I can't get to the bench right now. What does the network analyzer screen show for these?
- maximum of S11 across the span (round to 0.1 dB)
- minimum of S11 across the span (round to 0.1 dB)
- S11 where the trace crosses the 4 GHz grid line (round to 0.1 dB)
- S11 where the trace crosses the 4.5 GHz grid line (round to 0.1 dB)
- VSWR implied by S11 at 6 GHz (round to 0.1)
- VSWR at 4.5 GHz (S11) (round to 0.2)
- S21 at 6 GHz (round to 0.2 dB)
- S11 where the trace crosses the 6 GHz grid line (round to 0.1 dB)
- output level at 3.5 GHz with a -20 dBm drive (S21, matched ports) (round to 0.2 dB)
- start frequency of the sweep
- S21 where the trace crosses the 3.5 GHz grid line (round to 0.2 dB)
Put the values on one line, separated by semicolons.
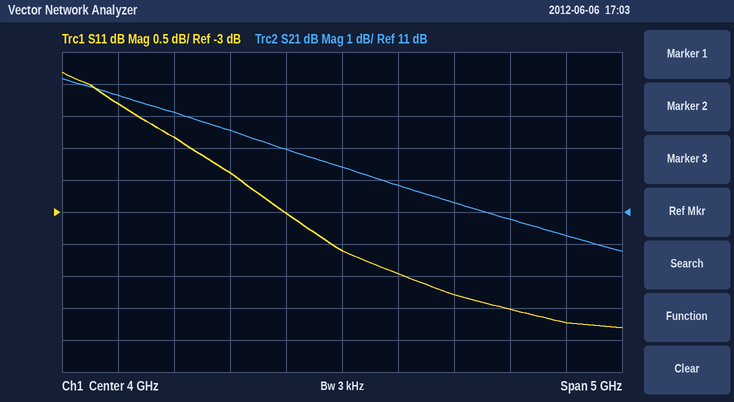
-0.8 dB; -4.8 dB; -3.6 dB; -4.0 dB; 3.8; 4.4; 10.2 dB; -4.7 dB; -7.0 dBm; 1.5 GHz; 13.0 dB
